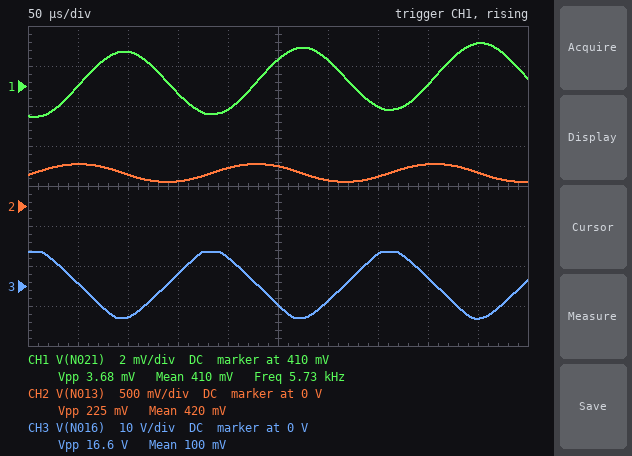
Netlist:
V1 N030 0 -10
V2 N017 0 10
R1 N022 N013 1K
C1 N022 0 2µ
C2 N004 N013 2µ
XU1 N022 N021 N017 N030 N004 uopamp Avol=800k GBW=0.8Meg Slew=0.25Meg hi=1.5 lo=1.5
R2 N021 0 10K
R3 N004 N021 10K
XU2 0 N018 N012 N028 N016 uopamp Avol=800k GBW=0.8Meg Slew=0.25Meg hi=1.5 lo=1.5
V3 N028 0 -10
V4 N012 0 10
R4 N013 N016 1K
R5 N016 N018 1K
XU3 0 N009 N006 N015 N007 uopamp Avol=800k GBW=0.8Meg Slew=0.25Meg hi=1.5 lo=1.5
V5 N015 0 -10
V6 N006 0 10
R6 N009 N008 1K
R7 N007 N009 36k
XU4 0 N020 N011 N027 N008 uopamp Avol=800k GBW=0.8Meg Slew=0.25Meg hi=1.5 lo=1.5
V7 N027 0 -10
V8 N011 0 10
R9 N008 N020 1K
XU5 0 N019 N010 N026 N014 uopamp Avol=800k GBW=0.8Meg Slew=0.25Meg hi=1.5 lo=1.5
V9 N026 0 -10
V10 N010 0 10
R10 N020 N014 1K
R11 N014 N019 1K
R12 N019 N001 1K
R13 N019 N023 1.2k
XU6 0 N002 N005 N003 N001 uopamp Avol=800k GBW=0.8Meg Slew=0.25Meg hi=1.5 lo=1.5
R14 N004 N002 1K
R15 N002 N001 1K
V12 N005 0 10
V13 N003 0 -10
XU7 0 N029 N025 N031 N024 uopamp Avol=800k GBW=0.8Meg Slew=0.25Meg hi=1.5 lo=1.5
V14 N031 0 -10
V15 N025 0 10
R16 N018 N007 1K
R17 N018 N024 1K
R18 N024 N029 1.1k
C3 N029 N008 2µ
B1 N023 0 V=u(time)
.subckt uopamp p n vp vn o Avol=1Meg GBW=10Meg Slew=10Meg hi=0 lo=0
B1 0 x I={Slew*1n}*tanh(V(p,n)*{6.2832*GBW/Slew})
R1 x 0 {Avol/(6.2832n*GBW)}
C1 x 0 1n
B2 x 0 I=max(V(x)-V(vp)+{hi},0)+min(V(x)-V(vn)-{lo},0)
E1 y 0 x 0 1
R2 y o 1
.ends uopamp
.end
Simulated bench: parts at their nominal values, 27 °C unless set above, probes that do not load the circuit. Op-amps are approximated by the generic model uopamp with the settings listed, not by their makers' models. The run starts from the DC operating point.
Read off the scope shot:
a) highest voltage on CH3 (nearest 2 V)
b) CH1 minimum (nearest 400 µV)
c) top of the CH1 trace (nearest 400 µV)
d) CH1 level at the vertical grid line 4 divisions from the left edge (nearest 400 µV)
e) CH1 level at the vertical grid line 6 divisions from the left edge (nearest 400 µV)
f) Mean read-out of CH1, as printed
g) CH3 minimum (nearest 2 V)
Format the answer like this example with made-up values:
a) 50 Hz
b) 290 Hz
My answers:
a) 8 V
b) 408.4 mV
c) 412.0 mV
d) 408.8 mV
e) 411.2 mV
f) 410 mV
g) -8 V
